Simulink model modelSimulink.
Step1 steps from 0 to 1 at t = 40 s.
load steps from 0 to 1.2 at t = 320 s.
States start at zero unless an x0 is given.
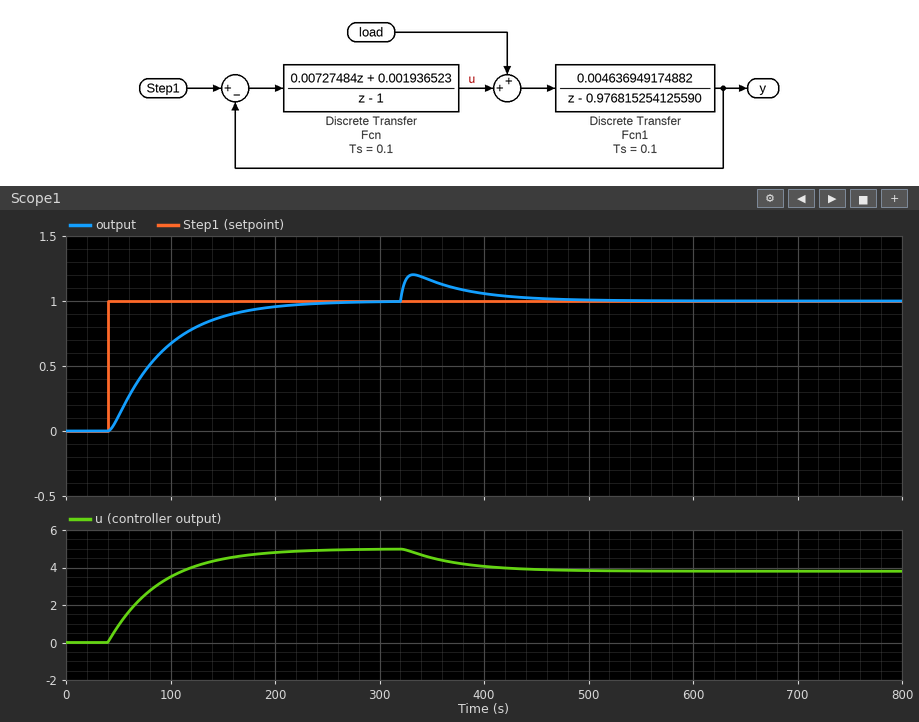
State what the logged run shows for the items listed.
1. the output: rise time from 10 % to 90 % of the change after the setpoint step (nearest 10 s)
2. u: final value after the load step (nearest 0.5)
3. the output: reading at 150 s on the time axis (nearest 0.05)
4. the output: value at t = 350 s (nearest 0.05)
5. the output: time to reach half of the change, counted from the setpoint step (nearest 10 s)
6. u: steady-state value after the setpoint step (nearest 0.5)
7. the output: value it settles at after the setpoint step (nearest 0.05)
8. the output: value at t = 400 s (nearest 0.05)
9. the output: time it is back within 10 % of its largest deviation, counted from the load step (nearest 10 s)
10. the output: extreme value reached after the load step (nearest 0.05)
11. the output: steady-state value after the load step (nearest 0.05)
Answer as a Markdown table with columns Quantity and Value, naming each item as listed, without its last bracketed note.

| Quantity | Value |
|---|---|
| the output: rise time from 10 % to 90 % of the change after the setpoint step | 110 s |
| u: final value after the load step | 4.0 |
| the output: reading at 150 s on the time axis | 0.90 |
| the output: value at t = 350 s | 1.15 |
| the output: time to reach half of the change, counted from the setpoint step | 40 s |
| u: steady-state value after the setpoint step | 5.0 |
| the output: value it settles at after the setpoint step | 1.00 |
| the output: value at t = 400 s | 1.05 |
| the output: time it is back within 10 % of its largest deviation, counted from the load step | 130 s |
| the output: extreme value reached after the load step | 1.20 |
| the output: steady-state value after the load step | 1.00 |
